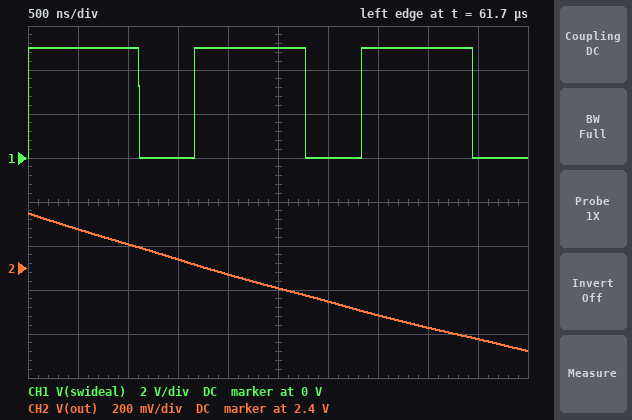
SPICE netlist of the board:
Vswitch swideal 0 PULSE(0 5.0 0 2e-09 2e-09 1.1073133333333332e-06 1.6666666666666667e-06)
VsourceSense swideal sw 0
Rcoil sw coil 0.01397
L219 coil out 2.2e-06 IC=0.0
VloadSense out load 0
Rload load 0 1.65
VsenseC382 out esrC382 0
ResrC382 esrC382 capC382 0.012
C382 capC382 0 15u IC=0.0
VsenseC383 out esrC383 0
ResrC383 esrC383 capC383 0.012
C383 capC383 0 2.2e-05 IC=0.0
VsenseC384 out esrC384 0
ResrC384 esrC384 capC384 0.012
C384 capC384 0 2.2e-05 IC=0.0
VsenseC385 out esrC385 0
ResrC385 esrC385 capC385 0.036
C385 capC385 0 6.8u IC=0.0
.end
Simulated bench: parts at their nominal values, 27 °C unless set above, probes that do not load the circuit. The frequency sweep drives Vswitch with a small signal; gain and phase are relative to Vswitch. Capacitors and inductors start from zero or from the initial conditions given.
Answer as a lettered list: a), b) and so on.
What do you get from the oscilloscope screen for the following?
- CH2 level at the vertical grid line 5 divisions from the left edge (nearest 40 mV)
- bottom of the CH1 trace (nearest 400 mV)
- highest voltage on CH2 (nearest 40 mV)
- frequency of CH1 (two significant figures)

a) 2.32 V
b) 0 V
c) 2.64 V
d) 600 kHz
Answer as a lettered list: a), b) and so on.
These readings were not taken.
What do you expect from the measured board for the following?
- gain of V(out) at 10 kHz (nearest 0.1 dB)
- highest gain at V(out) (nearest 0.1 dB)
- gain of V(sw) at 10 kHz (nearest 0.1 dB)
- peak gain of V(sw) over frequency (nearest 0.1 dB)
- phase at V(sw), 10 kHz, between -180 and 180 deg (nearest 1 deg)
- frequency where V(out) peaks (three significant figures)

a) 6.7 dB
b) 13.7 dB
c) 0 dB
d) 0 dB
e) 0 deg
f) 13.1 kHz
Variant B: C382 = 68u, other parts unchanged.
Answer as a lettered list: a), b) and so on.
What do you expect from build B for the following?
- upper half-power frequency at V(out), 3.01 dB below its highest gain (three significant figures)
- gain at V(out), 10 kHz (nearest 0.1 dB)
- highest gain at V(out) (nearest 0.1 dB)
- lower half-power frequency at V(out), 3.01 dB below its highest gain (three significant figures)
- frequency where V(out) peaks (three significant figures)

a) 10.8 kHz
b) 12.9 dB
c) 13.1 dB
d) 8.59 kHz
e) 9.75 kHz
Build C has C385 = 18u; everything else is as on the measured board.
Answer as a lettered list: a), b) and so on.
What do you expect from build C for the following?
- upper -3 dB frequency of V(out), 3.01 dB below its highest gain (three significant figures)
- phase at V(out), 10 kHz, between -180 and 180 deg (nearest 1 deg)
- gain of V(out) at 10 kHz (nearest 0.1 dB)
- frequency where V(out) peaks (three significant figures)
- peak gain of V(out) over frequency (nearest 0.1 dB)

a) 13.4 kHz
b) -26 deg
c) 8.4 dB
d) 12.1 kHz
e) 13.5 dB
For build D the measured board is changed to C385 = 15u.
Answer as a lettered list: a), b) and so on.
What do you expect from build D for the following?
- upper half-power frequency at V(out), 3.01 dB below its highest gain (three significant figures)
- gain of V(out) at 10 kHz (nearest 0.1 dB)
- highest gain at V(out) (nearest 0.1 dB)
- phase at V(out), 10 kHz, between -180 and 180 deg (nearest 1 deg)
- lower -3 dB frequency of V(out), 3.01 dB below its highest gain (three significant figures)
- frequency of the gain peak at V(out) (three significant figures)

a) 13.6 kHz
b) 7.9 dB
c) 13.6 dB
d) -24 deg
e) 11.0 kHz
f) 12.4 kHz
